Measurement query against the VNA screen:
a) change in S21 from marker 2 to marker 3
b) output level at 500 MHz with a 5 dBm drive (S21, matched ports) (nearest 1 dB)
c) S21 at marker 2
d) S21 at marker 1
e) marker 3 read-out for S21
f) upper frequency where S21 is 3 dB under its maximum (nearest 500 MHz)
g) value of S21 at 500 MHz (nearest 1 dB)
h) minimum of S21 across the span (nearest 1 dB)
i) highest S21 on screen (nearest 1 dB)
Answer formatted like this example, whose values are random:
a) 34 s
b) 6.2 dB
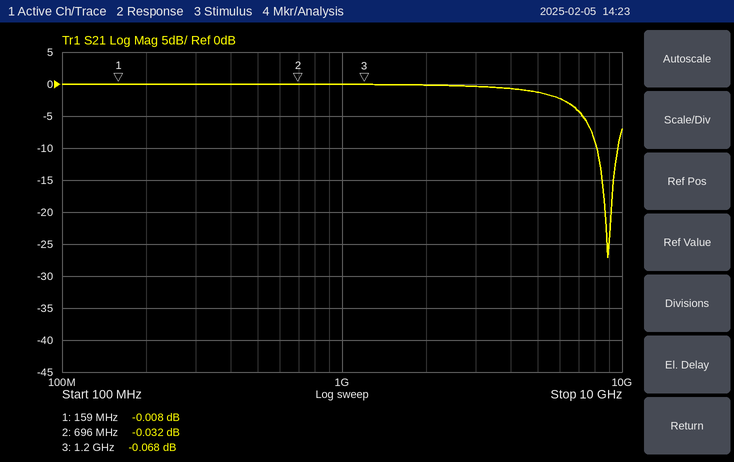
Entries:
a) -0.036 dB
b) 5 dBm
c) -0.032 dB
d) -0.008 dB
e) -0.068 dB
f) 6.5 GHz
g) 0 dB
h) -27 dB
i) 0 dB
